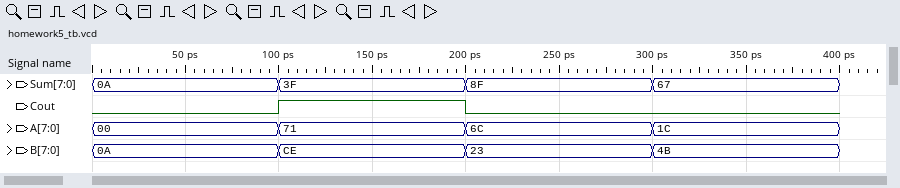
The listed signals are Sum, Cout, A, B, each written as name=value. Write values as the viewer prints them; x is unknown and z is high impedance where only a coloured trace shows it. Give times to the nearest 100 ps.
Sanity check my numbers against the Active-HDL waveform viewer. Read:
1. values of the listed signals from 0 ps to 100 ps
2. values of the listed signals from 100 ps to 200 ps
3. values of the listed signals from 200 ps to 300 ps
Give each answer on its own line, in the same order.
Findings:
Sum=0A, Cout=0, A=00, B=0A
Sum=3F, Cout=1, A=71, B=CE
Sum=8F, Cout=0, A=6C, B=23
